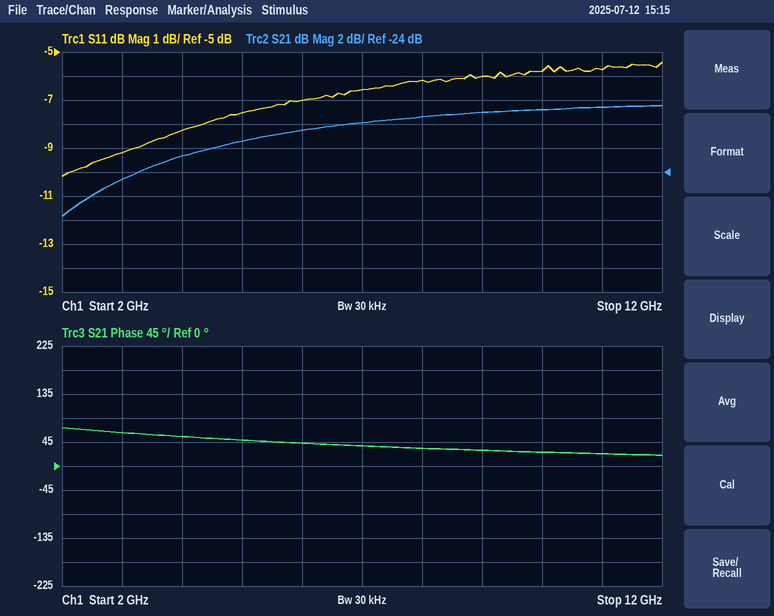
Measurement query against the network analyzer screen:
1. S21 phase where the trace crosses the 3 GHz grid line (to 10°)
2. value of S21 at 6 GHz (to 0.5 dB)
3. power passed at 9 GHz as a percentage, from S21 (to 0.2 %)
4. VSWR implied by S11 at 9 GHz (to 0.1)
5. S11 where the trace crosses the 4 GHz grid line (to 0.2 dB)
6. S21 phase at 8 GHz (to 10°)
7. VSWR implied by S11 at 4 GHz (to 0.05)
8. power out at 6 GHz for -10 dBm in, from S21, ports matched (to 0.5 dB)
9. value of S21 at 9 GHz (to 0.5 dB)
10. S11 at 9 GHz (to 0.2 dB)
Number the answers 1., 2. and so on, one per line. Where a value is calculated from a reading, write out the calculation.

1. 60°
2. -20.5 dB
3. 10^(-19/10) ≈ 1.26 %, so 1.2 % to the nearest 0.2 %
4. |Γ| = 10^(-6/20) = 0.5012; VSWR = (1 + 0.5012)/(1 − 0.5012) ≈ 3.0
5. -8.2 dB
6. 30°
7. |Γ| = 10^(-8.2/20) = 0.3890; VSWR = (1 + 0.3890)/(1 − 0.3890) ≈ 2.27, so 2.25 to the nearest 0.05
8. -10 dBm + (-20.5 dB) = -30.5 dBm
9. -19.0 dB
10. -6.0 dB
